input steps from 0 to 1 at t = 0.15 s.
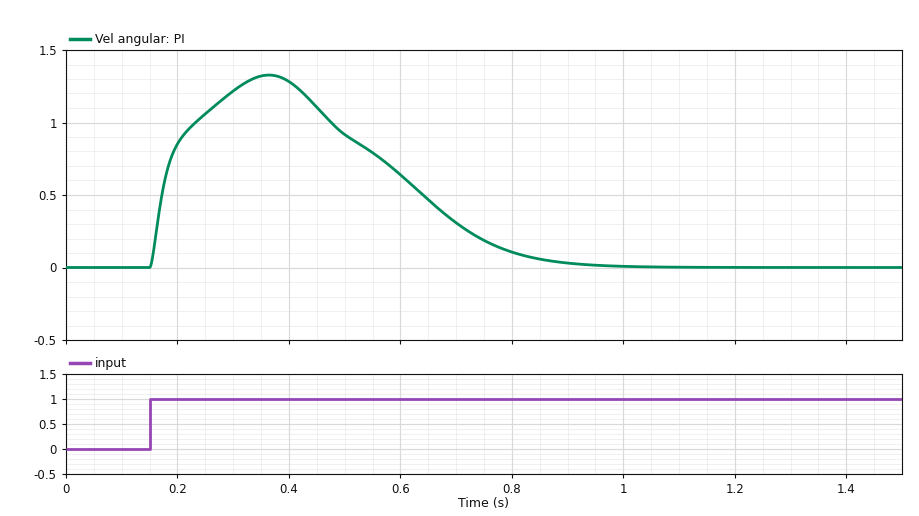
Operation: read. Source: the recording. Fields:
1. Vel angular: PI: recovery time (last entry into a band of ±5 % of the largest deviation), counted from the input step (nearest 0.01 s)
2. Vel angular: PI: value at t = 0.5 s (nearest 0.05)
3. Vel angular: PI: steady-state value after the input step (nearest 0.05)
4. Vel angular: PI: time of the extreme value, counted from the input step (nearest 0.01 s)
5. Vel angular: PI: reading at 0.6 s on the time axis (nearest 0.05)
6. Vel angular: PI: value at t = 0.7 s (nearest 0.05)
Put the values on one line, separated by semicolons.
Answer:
0.69 s; 0.90; 0.00; 0.21 s; 0.65; 0.30
